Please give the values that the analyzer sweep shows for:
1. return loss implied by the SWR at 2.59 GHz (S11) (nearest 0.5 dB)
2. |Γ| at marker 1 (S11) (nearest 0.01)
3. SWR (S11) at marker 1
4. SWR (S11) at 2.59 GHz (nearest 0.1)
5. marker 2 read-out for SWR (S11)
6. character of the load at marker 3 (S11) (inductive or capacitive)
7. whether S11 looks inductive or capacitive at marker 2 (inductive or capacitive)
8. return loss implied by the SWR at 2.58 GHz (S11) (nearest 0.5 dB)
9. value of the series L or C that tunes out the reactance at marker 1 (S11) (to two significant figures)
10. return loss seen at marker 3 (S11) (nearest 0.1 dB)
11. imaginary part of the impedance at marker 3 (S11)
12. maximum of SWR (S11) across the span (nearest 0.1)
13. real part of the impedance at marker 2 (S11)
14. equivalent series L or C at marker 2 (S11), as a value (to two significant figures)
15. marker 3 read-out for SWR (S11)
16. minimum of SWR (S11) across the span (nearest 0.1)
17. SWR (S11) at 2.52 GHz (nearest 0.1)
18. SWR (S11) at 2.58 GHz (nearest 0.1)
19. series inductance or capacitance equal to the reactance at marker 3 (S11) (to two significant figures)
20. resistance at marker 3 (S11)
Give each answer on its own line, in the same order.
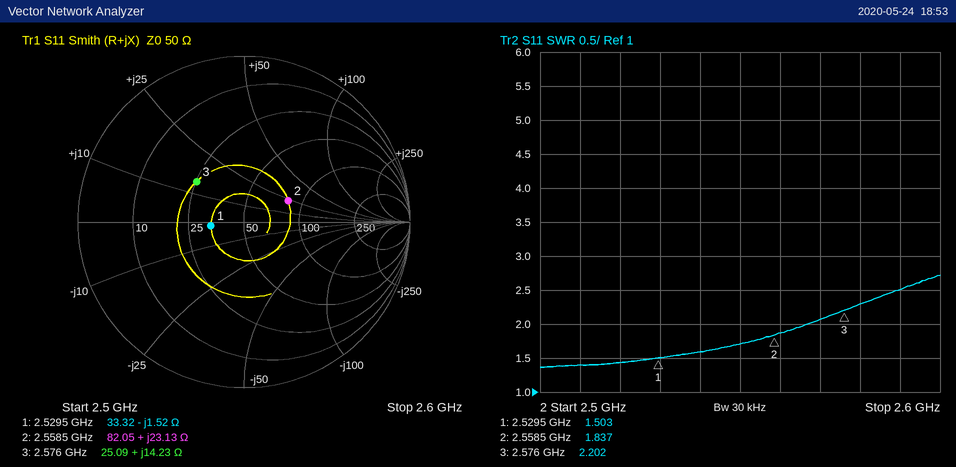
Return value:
7.5 dB
0.20
1.503
2.5
1.837
inductive
inductive
8.0 dB
96 pH
8.5 dB
+14.23 Ω
2.7
82.05 Ω
1.4 nH
2.202
1.4
1.4
2.3
880 pH
25.09 Ω
